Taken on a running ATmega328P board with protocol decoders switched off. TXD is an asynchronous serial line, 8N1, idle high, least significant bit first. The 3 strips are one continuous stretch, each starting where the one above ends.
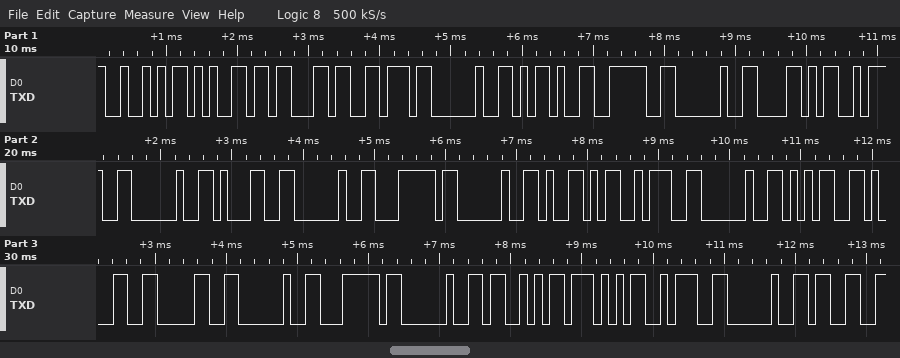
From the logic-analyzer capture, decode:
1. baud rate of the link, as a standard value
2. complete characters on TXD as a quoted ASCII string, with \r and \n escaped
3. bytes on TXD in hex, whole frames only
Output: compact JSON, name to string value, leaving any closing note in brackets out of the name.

{"baud rate of the link, as a standard value": "9600 baud", "complete characters on TXD as a quoted ASCII string, with \\r and \\n escaped": "\"Recv -> X: 1 | Y: 510 | SW: 3\"", "bytes on TXD in hex, whole frames only": "52 65 63 76 20 2D 3E 20 58 3A 20 31 20 7C 20 59 3A 20 35 31 30 20 7C 20 53 57 3A 20 33"}
